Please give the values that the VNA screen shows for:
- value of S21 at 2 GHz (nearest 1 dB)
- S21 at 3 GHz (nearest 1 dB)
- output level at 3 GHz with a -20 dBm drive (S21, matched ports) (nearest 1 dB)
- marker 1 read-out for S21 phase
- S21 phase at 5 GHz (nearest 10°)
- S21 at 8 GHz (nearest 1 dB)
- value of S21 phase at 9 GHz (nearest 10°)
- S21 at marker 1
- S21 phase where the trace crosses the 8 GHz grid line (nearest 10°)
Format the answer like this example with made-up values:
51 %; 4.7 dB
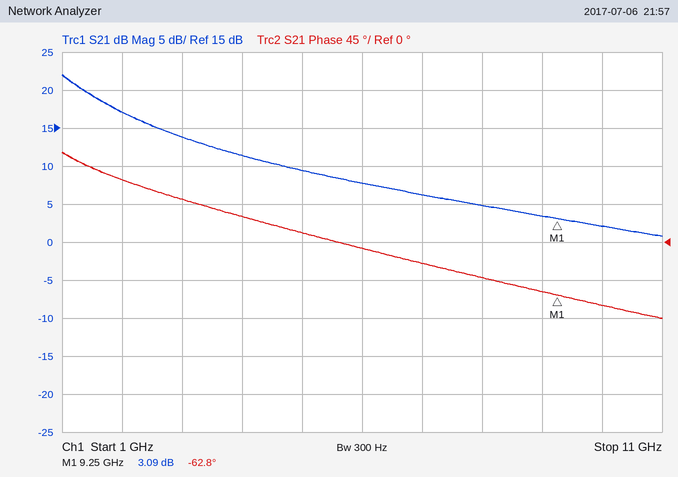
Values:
17 dB; 14 dB; -6 dBm; -62.8°; 10°; 5 dB; -60°; 3.09 dB; -40°
